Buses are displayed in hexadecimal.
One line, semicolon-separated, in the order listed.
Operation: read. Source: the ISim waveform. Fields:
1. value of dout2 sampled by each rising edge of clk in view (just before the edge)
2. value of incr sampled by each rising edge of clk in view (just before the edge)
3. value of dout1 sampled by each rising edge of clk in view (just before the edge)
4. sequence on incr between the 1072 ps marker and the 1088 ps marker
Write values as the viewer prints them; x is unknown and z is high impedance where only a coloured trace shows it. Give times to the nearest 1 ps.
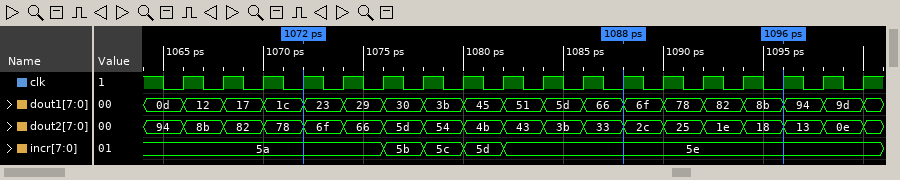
94, 8b, 82, 78, 6f, 66, 5d, 54, 4b, 43, 3b, 33, 2c, 25, 1e, 18, 13, 0e; 5a, 5a, 5a, 5a, 5a, 5a, 5b, 5c, 5d, 5e, 5e, 5e, 5e, 5e, 5e, 5e, 5e, 5e; 0d, 12, 17, 1c, 23, 29, 30, 3b, 45, 51, 5d, 66, 6f, 78, 82, 8b, 94, 9d; 5a, 5b, 5c, 5d, 5e
